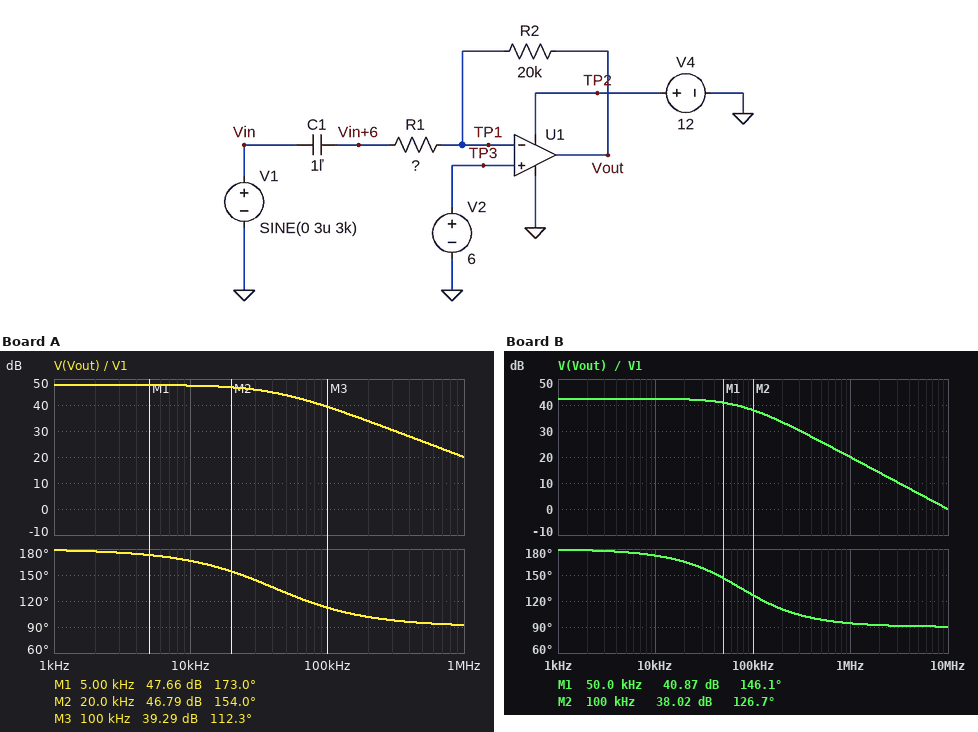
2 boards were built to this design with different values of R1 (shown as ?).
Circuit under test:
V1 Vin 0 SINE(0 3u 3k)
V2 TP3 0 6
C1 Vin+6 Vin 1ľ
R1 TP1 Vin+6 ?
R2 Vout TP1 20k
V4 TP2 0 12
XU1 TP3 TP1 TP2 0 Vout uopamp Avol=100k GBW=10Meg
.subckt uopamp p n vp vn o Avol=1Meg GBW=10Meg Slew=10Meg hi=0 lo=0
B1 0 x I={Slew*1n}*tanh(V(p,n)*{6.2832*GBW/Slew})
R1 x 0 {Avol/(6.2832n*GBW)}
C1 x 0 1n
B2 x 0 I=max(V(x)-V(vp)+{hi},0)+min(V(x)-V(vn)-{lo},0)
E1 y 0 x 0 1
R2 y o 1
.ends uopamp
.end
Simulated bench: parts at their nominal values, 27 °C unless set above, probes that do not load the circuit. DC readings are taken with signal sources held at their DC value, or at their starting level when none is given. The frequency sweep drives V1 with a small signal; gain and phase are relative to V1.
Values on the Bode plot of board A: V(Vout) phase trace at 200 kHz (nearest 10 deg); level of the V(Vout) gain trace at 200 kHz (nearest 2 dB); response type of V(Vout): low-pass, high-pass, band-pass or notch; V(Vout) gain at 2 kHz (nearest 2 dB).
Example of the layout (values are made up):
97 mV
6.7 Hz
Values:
100 deg
34 dB
low-pass
48 dB
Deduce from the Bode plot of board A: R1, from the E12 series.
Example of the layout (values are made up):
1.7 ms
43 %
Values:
82 Ω
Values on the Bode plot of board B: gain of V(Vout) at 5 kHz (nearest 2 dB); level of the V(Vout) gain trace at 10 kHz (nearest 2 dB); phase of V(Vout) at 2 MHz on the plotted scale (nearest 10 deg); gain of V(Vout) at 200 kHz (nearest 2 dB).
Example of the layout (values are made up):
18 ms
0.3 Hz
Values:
42 dB
42 dB
90 deg
34 dB
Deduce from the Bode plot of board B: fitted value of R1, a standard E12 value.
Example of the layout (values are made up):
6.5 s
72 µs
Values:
150 Ω
